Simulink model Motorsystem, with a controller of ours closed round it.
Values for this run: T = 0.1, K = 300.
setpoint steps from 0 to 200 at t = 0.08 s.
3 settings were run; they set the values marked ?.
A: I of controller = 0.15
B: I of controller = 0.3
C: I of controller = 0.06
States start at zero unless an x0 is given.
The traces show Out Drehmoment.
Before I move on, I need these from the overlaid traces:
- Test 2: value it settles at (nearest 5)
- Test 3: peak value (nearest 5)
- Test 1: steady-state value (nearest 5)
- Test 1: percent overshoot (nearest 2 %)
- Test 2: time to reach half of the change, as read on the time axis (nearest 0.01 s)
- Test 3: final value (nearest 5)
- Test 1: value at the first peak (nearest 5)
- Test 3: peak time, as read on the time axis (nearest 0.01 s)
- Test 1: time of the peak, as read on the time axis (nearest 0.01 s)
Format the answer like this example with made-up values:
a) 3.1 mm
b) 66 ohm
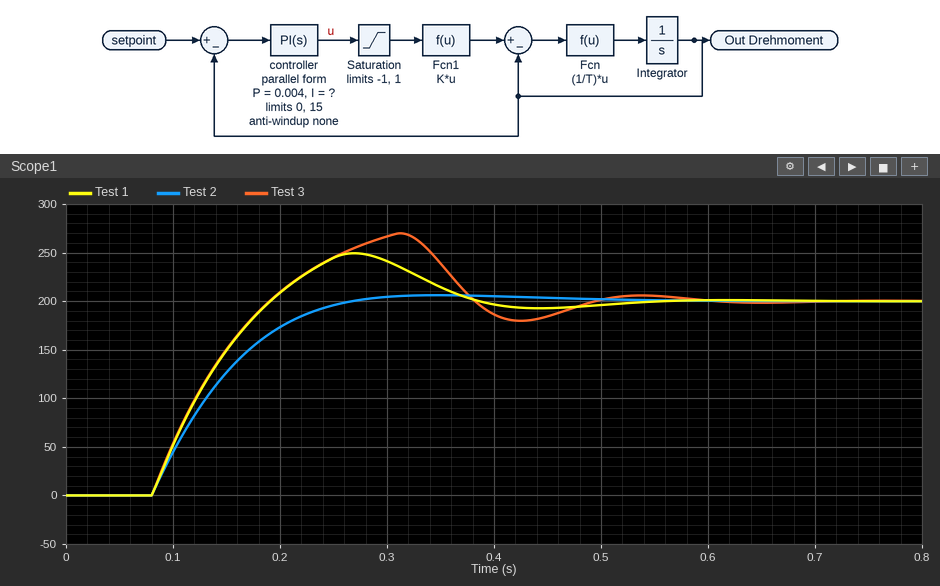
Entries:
a) 200
b) 270
c) 200
d) 24 %
e) 0.13 s
f) 200
g) 250
h) 0.31 s
i) 0.27 s
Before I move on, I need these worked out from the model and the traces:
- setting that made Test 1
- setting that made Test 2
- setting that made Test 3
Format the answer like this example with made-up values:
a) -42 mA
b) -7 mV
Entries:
a) A
b) C
c) B
